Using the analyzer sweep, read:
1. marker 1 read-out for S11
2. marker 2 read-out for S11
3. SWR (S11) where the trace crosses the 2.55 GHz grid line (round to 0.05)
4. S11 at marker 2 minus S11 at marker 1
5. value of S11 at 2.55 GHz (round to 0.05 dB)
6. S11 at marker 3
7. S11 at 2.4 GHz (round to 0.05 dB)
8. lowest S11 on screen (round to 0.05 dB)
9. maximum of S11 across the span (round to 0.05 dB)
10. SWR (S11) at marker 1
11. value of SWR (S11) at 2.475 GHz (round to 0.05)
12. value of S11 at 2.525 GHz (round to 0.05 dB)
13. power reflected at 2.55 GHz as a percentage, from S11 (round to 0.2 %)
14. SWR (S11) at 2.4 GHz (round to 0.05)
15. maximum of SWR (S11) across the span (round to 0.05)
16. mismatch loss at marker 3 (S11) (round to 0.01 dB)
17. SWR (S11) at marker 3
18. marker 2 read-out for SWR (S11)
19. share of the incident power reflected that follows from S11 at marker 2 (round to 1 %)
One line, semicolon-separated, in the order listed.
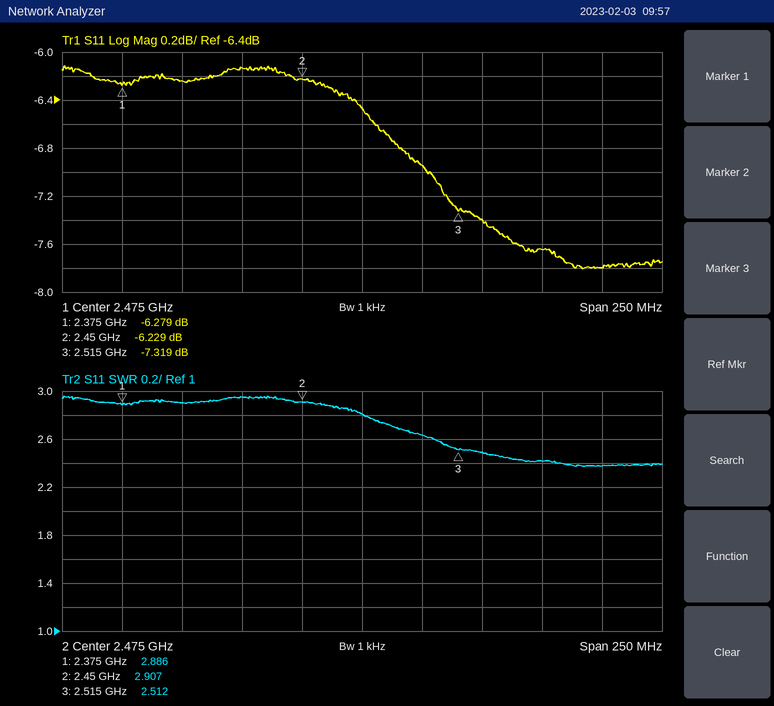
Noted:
-6.279 dB; -6.229 dB; 2.40; 0.050 dB; -7.65 dB; -7.319 dB; -6.25 dB; -7.80 dB; -6.10 dB; 2.886; 2.80; -7.40 dB; 17.2 %; 2.90; 2.95; 0.89 dB; 2.512; 2.907; 24 %
